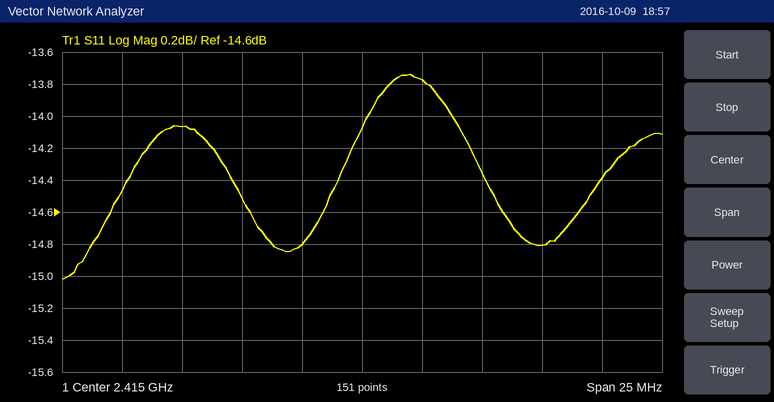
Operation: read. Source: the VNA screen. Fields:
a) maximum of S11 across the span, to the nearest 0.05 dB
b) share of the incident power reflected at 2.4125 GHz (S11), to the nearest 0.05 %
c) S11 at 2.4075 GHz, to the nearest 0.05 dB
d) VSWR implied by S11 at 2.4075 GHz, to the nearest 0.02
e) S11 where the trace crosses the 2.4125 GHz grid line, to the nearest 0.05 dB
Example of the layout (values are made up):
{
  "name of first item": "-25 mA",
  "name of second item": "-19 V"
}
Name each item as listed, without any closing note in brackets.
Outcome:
{
  "maximum of S11 across the span, to the nearest 0.05 dB": "-13.75 dB",
  "share of the incident power reflected at 2.4125 GHz (S11), to the nearest 0.05 %": "3.30 %",
  "S11 at 2.4075 GHz, to the nearest 0.05 dB": "-14.05 dB",
  "VSWR implied by S11 at 2.4075 GHz, to the nearest 0.02": "1.50",
  "S11 where the trace crosses the 2.4125 GHz grid line, to the nearest 0.05 dB": "-14.80 dB"
}
